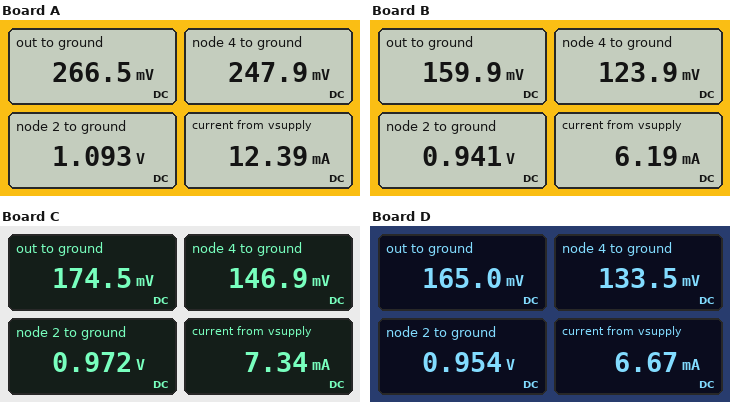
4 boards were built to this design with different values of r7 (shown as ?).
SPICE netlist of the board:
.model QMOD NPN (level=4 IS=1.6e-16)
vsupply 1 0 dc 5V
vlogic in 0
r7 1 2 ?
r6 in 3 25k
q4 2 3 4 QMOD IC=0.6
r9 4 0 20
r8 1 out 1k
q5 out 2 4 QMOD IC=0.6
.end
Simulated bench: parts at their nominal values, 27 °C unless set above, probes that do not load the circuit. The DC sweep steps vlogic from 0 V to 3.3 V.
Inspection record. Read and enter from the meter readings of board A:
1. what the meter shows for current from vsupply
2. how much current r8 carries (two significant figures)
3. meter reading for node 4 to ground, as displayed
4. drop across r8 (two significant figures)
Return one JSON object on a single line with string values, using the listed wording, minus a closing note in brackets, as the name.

{"what the meter shows for current from vsupply": "12.39 mA", "how much current r8 carries": "4.7 mA", "meter reading for node 4 to ground, as displayed": "247.9 mV", "drop across r8": "4.7 V"}
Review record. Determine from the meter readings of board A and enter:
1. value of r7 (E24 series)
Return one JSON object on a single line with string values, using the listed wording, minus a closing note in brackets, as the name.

{"value of r7": "510 Ω"}
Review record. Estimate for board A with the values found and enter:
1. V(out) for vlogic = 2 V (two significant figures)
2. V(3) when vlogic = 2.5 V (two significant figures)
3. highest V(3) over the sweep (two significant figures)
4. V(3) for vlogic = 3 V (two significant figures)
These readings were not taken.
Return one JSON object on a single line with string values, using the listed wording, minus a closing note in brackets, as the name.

{"V(out) for vlogic = 2 V": "280 mV", "V(3) when vlogic = 2.5 V": "1.0 V", "highest V(3) over the sweep": "1.1 V", "V(3) for vlogic = 3 V": "1.0 V"}
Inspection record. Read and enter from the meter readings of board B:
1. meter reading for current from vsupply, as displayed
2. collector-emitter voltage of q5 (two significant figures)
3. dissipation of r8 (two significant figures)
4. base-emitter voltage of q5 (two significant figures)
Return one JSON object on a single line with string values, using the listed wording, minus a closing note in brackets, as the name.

{"meter reading for current from vsupply, as displayed": "6.19 mA", "collector-emitter voltage of q5": "36 mV", "dissipation of r8": "23 mW", "base-emitter voltage of q5": "820 mV"}
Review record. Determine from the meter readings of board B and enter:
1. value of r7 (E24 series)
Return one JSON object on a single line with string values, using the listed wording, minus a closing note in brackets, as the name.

{"value of r7": "3 kΩ"}
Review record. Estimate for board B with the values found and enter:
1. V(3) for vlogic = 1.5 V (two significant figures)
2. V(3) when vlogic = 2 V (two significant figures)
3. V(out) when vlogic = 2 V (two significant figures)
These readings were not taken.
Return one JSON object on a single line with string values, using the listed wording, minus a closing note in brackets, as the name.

{"V(3) for vlogic = 1.5 V": "810 mV", "V(3) when vlogic = 2 V": "810 mV", "V(out) when vlogic = 2 V": "5.0 V"}
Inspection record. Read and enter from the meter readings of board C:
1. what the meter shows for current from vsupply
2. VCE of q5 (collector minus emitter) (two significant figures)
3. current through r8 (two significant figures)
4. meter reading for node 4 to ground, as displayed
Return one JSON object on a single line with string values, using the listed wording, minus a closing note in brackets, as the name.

{"what the meter shows for current from vsupply": "7.34 mA", "VCE of q5 (collector minus emitter)": "28 mV", "current through r8": "4.8 mA", "meter reading for node 4 to ground, as displayed": "146.9 mV"}
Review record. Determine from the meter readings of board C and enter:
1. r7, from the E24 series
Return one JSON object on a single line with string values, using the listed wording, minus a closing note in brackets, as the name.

{"r7, from the E24 series": "1.6 kΩ"}
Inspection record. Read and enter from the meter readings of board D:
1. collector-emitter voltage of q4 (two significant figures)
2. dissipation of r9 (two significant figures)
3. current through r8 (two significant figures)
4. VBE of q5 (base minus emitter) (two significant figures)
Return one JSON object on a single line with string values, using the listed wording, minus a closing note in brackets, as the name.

{"collector-emitter voltage of q4": "820 mV", "dissipation of r9": "890 µW", "current through r8": "4.8 mA", "VBE of q5 (base minus emitter)": "820 mV"}
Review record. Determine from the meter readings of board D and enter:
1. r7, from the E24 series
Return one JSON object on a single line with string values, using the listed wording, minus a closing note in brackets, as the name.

{"r7, from the E24 series": "2.2 kΩ"}
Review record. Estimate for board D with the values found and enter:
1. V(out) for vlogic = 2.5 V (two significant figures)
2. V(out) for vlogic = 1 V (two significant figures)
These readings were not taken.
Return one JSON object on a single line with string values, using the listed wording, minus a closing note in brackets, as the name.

{"V(out) for vlogic = 2.5 V": "5.0 V", "V(out) for vlogic = 1 V": "170 mV"}
